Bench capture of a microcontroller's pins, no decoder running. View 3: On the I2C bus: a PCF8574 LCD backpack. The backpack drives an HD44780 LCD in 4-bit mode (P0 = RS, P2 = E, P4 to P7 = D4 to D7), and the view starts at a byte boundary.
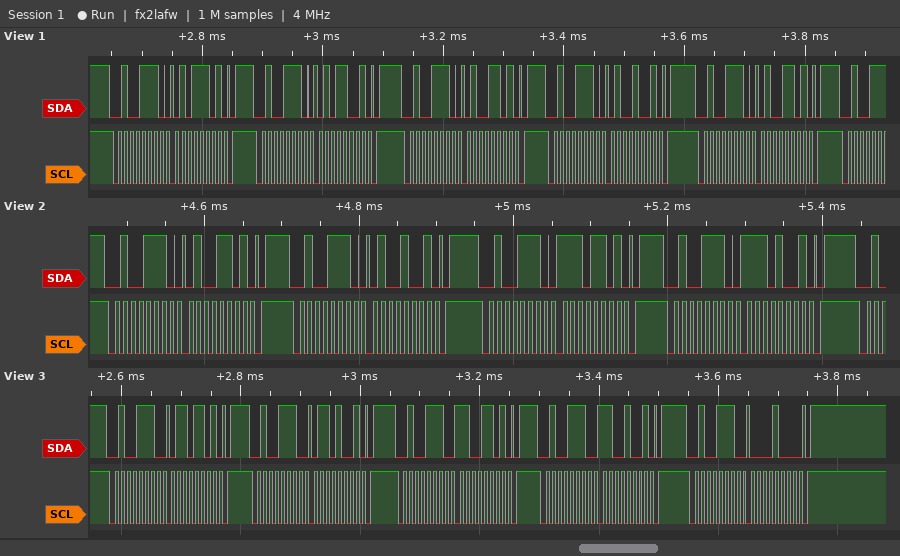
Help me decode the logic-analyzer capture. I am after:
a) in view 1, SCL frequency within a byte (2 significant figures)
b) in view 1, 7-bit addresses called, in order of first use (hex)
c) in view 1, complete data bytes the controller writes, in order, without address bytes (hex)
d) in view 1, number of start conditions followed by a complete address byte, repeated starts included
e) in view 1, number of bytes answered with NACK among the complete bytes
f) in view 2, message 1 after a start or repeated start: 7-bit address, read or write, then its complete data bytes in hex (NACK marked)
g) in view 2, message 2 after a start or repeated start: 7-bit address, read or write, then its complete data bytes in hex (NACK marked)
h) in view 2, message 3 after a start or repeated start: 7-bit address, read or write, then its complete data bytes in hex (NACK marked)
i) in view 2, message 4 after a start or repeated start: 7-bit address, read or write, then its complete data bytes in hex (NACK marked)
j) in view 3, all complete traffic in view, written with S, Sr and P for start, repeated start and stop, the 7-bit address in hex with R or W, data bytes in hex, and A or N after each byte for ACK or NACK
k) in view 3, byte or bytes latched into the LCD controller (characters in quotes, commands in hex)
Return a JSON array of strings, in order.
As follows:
["100 kHz", "0x27", "5D 59 4D 49 4D", "5", "0", "0x27 write: 4D", "0x27 write: 49", "0x27 write: ED", "0x27 write: E9", "S 27W A 6D A P S 27W A 69 A P S 27W A CD A P S 27W A C9 A P S 27W A 08 A P", "'l'"]
